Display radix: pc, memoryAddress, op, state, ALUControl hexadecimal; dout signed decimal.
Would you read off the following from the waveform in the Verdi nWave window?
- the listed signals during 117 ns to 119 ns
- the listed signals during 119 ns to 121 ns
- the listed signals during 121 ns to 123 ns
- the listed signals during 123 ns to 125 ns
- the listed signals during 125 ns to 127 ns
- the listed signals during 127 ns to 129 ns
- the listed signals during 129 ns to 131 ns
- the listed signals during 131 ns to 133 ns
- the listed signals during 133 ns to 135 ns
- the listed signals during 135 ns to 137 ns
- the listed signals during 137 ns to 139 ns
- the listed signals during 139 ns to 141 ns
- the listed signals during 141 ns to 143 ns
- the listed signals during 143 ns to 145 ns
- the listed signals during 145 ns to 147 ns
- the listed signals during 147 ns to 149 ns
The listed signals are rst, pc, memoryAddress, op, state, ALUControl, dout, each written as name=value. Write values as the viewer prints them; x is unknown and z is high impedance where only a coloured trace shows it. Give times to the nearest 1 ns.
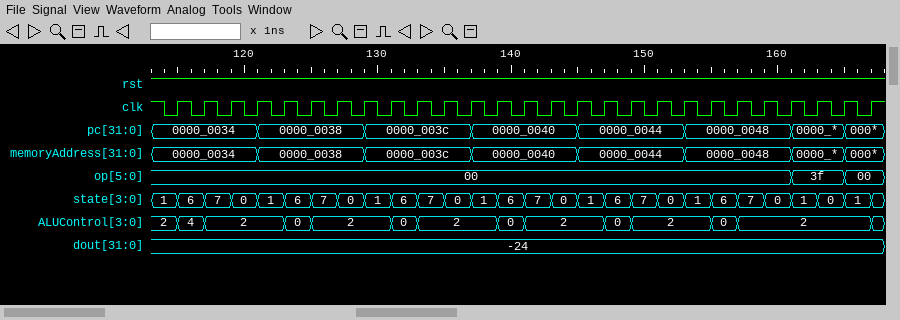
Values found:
rst=1, pc=0000_0034, memoryAddress=0000_0034, op=00, state=7, ALUControl=2, dout=-24
rst=1, pc=0000_0034, memoryAddress=0000_0034, op=00, state=0, ALUControl=2, dout=-24
rst=1, pc=0000_0038, memoryAddress=0000_0038, op=00, state=1, ALUControl=2, dout=-24
rst=1, pc=0000_0038, memoryAddress=0000_0038, op=00, state=6, ALUControl=0, dout=-24
rst=1, pc=0000_0038, memoryAddress=0000_0038, op=00, state=7, ALUControl=2, dout=-24
rst=1, pc=0000_0038, memoryAddress=0000_0038, op=00, state=0, ALUControl=2, dout=-24
rst=1, pc=0000_003c, memoryAddress=0000_003c, op=00, state=1, ALUControl=2, dout=-24
rst=1, pc=0000_003c, memoryAddress=0000_003c, op=00, state=6, ALUControl=0, dout=-24
rst=1, pc=0000_003c, memoryAddress=0000_003c, op=00, state=7, ALUControl=2, dout=-24
rst=1, pc=0000_003c, memoryAddress=0000_003c, op=00, state=0, ALUControl=2, dout=-24
rst=1, pc=0000_0040, memoryAddress=0000_0040, op=00, state=1, ALUControl=2, dout=-24
rst=1, pc=0000_0040, memoryAddress=0000_0040, op=00, state=6, ALUControl=0, dout=-24
rst=1, pc=0000_0040, memoryAddress=0000_0040, op=00, state=7, ALUControl=2, dout=-24
rst=1, pc=0000_0040, memoryAddress=0000_0040, op=00, state=0, ALUControl=2, dout=-24
rst=1, pc=0000_0044, memoryAddress=0000_0044, op=00, state=1, ALUControl=2, dout=-24
rst=1, pc=0000_0044, memoryAddress=0000_0044, op=00, state=6, ALUControl=0, dout=-24
